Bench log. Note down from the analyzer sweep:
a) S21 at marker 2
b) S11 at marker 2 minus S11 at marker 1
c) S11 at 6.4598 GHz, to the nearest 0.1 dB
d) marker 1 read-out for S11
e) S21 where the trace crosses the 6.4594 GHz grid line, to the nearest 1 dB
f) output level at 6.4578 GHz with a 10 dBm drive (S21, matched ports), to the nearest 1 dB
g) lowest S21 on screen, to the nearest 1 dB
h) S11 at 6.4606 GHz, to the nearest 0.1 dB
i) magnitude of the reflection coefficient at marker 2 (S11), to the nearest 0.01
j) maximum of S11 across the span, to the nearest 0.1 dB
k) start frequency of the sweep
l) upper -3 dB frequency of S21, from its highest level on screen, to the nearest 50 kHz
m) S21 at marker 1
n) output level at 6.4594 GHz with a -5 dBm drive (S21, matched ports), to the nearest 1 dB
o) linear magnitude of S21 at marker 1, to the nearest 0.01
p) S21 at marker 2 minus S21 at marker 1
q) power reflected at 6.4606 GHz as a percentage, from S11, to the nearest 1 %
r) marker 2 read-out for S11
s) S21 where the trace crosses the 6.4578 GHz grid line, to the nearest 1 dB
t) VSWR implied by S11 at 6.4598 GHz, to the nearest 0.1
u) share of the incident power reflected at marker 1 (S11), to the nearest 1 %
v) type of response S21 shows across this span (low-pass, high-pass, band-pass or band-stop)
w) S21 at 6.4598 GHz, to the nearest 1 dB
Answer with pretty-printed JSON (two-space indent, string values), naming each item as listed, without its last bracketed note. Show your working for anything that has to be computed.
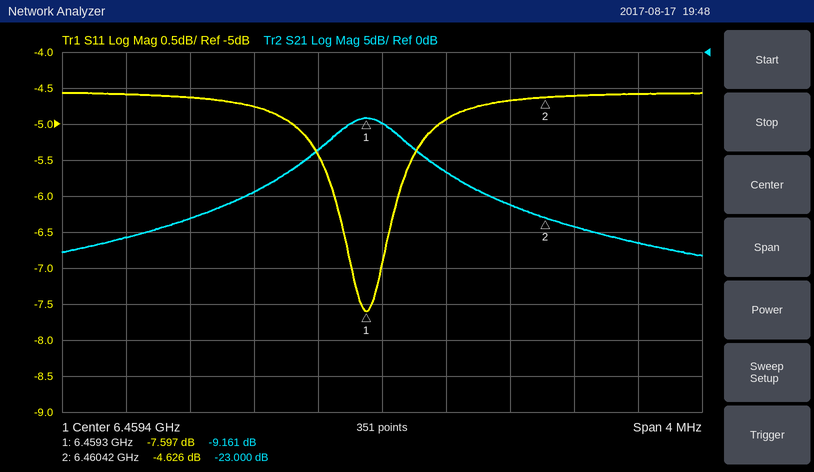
{
  "S21 at marker 2": "-23.000 dB",
  "S11 at marker 2 minus S11 at marker 1": "-4.626 − (-7.597) = 2.971 dB",
  "S11 at 6.4598 GHz, to the nearest 0.1 dB": "-4.9 dB",
  "marker 1 read-out for S11": "-7.597 dB",
  "S21 where the trace crosses the 6.4594 GHz grid line, to the nearest 1 dB": "-10 dB",
  "output level at 6.4578 GHz with a 10 dBm drive (S21, matched ports), to the nearest 1 dB": "10 dBm + (-26 dB) = -16 dBm",
  "lowest S21 on screen, to the nearest 1 dB": "-28 dB",
  "S11 at 6.4606 GHz, to the nearest 0.1 dB": "-4.6 dB",
  "magnitude of the reflection coefficient at marker 2 (S11), to the nearest 0.01": "10^(-4.626/20) ≈ 0.59",
  "maximum of S11 across the span, to the nearest 0.1 dB": "-4.6 dB",
  "start frequency of the sweep": "6.4574 GHz",
  "upper -3 dB frequency of S21, from its highest level on screen, to the nearest 50 kHz": "6.45955 GHz",
  "S21 at marker 1": "-9.161 dB",
  "output level at 6.4594 GHz with a -5 dBm drive (S21, matched ports), to the nearest 1 dB": "-5 dBm + (-10 dB) = -15 dBm",
  "linear magnitude of S21 at marker 1, to the nearest 0.01": "10^(-9.161/20) ≈ 0.35",
  "S21 at marker 2 minus S21 at marker 1": "-23 − (-9.161) = -13.839 dB",
  "power reflected at 6.4606 GHz as a percentage, from S11, to the nearest 1 %": "10^(-4.6/10) ≈ 35 %",
  "marker 2 read-out for S11": "-4.626 dB",
  "S21 where the trace crosses the 6.4578 GHz grid line, to the nearest 1 dB": "-26 dB",
  "VSWR implied by S11 at 6.4598 GHz, to the nearest 0.1": "|Γ| = 10^(-4.9/20) = 0.5689; VSWR = (1 + 0.5689)/(1 − 0.5689) ≈ 3.6",
  "share of the incident power reflected at marker 1 (S11), to the nearest 1 %": "10^(-7.597/10) ≈ 17 %",
  "type of response S21 shows across this span": "band-pass",
  "S21 at 6.4598 GHz, to the nearest 1 dB": "-17 dB"
}
